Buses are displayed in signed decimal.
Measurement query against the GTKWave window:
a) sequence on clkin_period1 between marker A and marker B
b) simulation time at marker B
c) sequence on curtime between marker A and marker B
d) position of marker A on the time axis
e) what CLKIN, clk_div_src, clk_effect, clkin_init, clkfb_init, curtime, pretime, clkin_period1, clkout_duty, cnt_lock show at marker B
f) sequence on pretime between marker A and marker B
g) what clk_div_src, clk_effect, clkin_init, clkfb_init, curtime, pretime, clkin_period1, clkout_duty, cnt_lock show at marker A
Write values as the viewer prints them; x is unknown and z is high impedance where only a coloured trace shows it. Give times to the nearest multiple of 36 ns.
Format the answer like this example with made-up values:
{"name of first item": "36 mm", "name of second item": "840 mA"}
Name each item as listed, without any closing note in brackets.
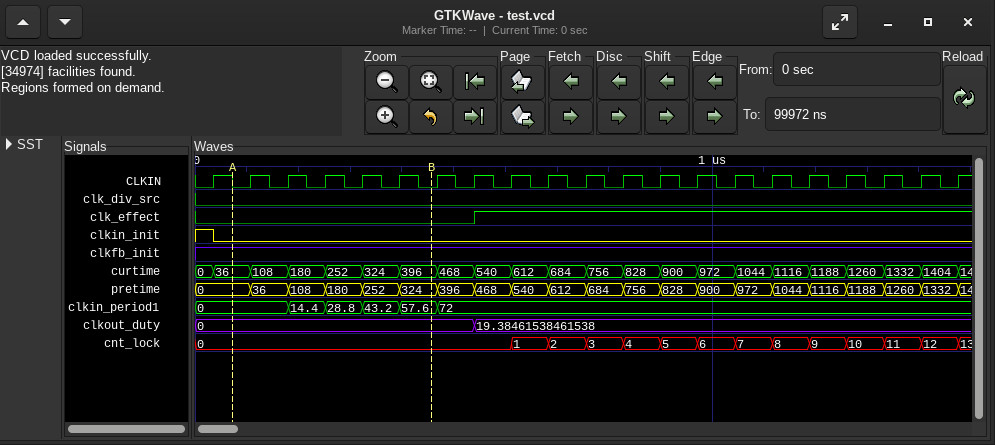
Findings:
{"sequence on clkin_period1 between marker A and marker B": "0, 14.4, 28.8, 43.2, 57.6", "simulation time at marker B": "468 ns", "sequence on curtime between marker A and marker B": "36, 108, 180, 252, 324, 396", "position of marker A on the time axis": "72 ns", "what CLKIN, clk_div_src, clk_effect, clkin_init, clkfb_init, curtime, pretime, clkin_period1, clkout_duty, cnt_lock show at marker B": "CLKIN=0, clk_div_src=0, clk_effect=0, clkin_init=0, clkfb_init=1, curtime=396, pretime=324, clkin_period1=57.6, clkout_duty=0, cnt_lock=0", "sequence on pretime between marker A and marker B": "0, 36, 108, 180, 252, 324", "what clk_div_src, clk_effect, clkin_init, clkfb_init, curtime, pretime, clkin_period1, clkout_duty, cnt_lock show at marker A": "clk_div_src=0, clk_effect=0, clkin_init=0, clkfb_init=1, curtime=36, pretime=0, clkin_period1=0, clkout_duty=0, cnt_lock=0"}
